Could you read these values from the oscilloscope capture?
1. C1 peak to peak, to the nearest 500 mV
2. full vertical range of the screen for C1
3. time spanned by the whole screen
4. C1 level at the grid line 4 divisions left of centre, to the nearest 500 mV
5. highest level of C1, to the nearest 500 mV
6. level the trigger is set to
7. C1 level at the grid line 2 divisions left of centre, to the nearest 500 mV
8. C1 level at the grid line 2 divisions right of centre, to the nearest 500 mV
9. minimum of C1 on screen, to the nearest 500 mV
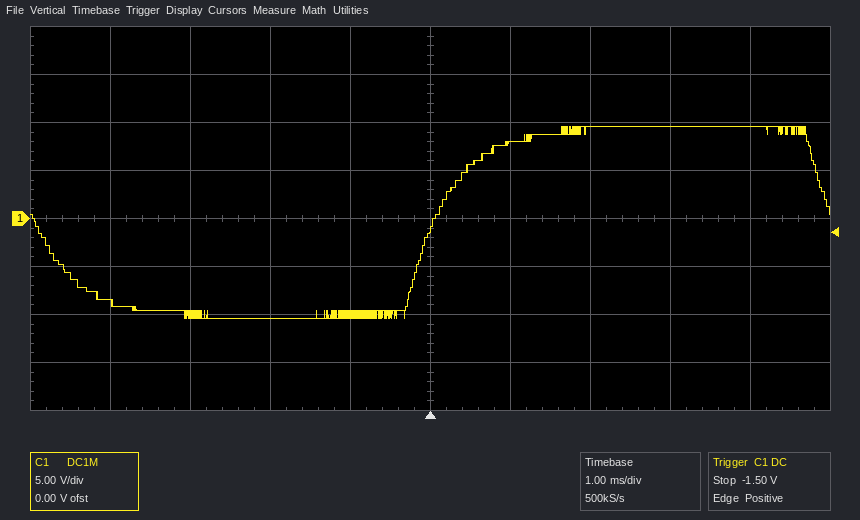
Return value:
20.0 V
40 V
10 ms
-9.0 V
9.5 V
-1.50 V
-10.5 V
9.5 V
-10.5 V
